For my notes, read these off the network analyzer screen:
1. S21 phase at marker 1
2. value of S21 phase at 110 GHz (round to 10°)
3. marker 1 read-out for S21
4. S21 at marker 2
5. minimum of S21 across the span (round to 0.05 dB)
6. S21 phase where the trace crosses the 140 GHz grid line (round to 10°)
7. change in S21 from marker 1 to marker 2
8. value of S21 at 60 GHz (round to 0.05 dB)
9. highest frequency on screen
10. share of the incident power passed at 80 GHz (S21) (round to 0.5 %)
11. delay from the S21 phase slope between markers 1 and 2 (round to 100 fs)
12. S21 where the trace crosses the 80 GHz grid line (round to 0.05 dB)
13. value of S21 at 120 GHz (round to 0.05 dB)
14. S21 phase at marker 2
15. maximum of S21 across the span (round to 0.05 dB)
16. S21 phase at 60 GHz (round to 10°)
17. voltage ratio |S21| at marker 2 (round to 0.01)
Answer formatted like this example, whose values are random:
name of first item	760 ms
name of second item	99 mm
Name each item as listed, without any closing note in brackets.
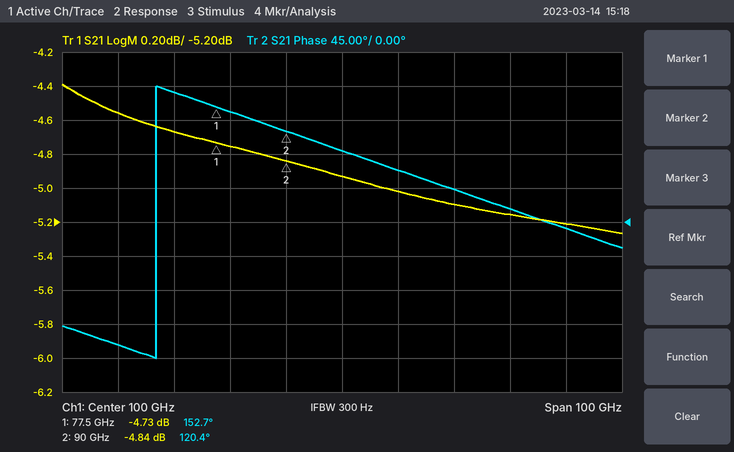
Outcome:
S21 phase at marker 1	152.7°
value of S21 phase at 110 GHz	70°
marker 1 read-out for S21	-4.73 dB
S21 at marker 2	-4.84 dB
minimum of S21 across the span	-5.25 dB
S21 phase where the trace crosses the 140 GHz grid line	-10°
change in S21 from marker 1 to marker 2	-0.11 dB
value of S21 at 60 GHz	-4.55 dB
highest frequency on screen	150 GHz
share of the incident power passed at 80 GHz (S21)	33.5 %
delay from the S21 phase slope between markers 1 and 2	7.2 ps
S21 where the trace crosses the 80 GHz grid line	-4.75 dB
value of S21 at 120 GHz	-5.10 dB
S21 phase at marker 2	120.4°
maximum of S21 across the span	-4.40 dB
S21 phase at 60 GHz	-160°
voltage ratio |S21| at marker 2	0.57
